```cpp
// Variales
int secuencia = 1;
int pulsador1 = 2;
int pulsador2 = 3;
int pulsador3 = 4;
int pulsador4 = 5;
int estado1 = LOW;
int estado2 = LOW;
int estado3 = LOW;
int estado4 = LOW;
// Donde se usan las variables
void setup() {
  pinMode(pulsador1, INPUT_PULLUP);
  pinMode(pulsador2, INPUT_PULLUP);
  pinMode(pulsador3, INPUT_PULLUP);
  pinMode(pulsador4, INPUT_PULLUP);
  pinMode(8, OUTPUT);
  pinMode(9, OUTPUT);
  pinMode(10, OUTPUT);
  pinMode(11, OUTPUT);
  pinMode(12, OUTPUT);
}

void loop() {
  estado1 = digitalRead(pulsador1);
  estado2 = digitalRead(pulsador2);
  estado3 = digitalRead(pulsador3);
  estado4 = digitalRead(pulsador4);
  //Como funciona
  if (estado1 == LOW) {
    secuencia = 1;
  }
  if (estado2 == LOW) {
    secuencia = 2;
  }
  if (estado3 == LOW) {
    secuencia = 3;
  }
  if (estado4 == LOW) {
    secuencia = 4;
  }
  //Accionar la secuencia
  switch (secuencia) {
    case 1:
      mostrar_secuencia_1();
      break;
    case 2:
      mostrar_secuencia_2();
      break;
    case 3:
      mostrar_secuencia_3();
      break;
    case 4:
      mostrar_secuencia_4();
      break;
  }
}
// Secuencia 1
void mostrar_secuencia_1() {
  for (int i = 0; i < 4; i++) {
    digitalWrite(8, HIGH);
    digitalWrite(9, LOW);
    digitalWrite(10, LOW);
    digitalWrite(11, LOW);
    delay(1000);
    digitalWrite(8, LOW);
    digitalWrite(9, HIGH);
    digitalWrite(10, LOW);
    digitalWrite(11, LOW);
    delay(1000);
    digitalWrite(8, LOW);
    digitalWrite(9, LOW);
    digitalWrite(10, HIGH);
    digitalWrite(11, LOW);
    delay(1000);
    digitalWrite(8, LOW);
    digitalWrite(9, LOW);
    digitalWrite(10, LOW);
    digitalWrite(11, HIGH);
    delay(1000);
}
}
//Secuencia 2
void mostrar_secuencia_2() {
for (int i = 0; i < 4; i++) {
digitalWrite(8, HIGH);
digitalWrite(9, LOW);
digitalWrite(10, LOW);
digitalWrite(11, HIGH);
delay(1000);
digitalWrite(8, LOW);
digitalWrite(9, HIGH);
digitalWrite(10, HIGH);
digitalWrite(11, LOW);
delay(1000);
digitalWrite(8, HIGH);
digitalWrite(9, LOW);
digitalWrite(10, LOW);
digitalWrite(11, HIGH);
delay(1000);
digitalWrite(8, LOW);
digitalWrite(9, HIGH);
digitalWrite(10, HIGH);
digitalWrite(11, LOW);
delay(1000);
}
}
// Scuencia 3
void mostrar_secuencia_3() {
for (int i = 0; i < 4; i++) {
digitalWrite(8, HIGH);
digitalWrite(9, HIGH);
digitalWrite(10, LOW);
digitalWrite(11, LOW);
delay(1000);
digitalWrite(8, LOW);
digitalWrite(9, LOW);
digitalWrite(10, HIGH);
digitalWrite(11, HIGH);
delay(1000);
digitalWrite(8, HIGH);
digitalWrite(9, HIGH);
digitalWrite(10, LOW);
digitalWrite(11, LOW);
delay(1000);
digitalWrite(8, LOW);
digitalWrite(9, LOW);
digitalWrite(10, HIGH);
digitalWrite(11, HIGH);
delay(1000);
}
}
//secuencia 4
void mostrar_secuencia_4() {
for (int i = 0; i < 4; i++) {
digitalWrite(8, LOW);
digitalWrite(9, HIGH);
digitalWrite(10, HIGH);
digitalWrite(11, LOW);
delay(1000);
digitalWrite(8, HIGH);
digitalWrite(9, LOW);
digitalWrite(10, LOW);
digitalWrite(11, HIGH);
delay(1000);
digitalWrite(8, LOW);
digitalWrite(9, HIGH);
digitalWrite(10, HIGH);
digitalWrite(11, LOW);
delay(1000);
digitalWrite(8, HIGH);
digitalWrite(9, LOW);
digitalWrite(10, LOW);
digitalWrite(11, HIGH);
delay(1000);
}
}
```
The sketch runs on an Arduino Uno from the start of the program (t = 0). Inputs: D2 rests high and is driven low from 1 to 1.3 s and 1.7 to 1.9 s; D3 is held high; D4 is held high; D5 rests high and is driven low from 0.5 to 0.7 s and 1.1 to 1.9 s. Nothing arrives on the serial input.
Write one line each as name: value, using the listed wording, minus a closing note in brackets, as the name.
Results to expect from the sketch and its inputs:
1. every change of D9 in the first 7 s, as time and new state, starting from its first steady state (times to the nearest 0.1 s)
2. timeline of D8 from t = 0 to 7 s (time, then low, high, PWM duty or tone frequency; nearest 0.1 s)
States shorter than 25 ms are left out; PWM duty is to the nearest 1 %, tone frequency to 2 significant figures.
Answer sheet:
every change of D9 in the first 7 s, as time and new state, starting from its first steady state: 0 s low; 1 s high; 2 s low; 5 s high; 6 s low
timeline of D8 from t = 0 to 7 s: 0 s high; 1 s low; 4 s high; 5 s low
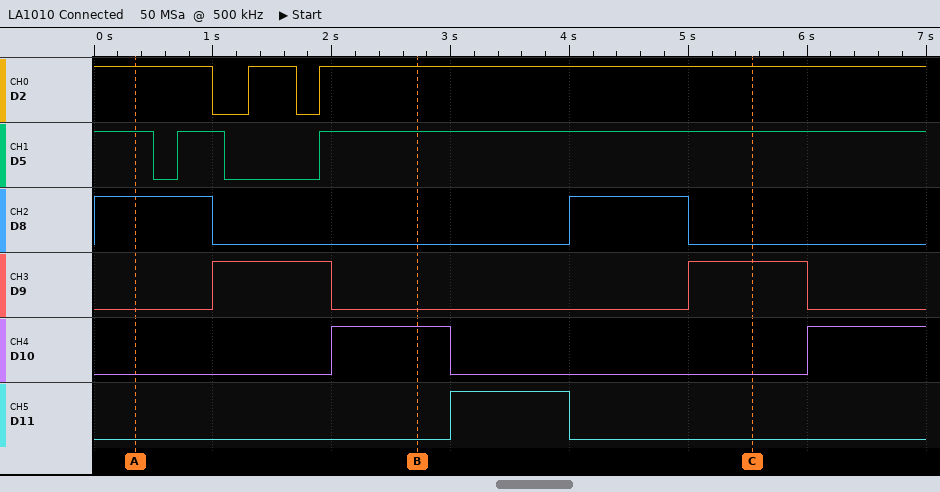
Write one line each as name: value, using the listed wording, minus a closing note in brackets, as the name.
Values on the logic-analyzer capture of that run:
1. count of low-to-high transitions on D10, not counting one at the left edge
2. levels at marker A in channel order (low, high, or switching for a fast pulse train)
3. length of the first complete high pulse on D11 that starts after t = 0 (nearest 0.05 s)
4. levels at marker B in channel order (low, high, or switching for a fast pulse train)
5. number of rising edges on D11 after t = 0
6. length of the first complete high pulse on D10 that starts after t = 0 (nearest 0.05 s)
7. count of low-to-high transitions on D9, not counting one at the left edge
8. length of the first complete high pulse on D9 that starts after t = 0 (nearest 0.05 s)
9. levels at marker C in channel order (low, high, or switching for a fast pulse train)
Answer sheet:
count of low-to-high transitions on D10, not counting one at the left edge: 2
levels at marker A in channel order: D2 high, D5 high, D8 high, D9 low, D10 low, D11 low
length of the first complete high pulse on D11 that starts after t = 0: 1.00 s
levels at marker B in channel order: D2 high, D5 high, D8 low, D9 low, D10 high, D11 low
number of rising edges on D11 after t = 0: 1
length of the first complete high pulse on D10 that starts after t = 0: 1.00 s
count of low-to-high transitions on D9, not counting one at the left edge: 2
length of the first complete high pulse on D9 that starts after t = 0: 1.00 s
levels at marker C in channel order: D2 high, D5 high, D8 low, D9 high, D10 low, D11 low
